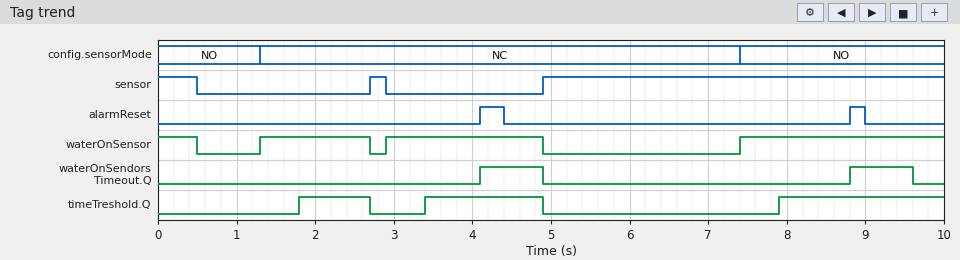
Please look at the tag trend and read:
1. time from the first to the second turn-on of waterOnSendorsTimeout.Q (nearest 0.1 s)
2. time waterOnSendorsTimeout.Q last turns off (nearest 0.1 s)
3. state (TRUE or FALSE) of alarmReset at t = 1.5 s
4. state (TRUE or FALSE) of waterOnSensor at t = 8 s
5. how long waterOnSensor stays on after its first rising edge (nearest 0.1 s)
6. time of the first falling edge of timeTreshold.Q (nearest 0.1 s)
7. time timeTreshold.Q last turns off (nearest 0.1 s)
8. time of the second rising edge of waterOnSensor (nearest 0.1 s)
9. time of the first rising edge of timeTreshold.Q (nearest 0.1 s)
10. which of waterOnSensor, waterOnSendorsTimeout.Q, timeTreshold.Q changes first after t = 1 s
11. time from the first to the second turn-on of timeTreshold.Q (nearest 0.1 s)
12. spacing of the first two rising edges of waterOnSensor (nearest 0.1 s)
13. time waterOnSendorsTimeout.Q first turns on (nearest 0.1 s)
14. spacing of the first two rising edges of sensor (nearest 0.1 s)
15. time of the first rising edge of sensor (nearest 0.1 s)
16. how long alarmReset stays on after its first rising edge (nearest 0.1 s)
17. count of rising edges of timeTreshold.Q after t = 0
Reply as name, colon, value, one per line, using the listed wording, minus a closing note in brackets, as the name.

time from the first to the second turn-on of waterOnSendorsTimeout.Q: 4.7 s
time waterOnSendorsTimeout.Q last turns off: 9.6 s
state (TRUE or FALSE) of alarmReset at t = 1.5 s: FALSE
state (TRUE or FALSE) of waterOnSensor at t = 8 s: TRUE
how long waterOnSensor stays on after its first rising edge: 1.4 s
time of the first falling edge of timeTreshold.Q: 2.7 s
time timeTreshold.Q last turns off: 4.9 s
time of the second rising edge of waterOnSensor: 2.9 s
time of the first rising edge of timeTreshold.Q: 1.8 s
which of waterOnSensor, waterOnSendorsTimeout.Q, timeTreshold.Q changes first after t = 1 s: waterOnSensor
time from the first to the second turn-on of timeTreshold.Q: 1.6 s
spacing of the first two rising edges of waterOnSensor: 1.6 s
time waterOnSendorsTimeout.Q first turns on: 4.1 s
spacing of the first two rising edges of sensor: 2.2 s
time of the first rising edge of sensor: 2.7 s
how long alarmReset stays on after its first rising edge: 0.3 s
count of rising edges of timeTreshold.Q after t = 0: 3
